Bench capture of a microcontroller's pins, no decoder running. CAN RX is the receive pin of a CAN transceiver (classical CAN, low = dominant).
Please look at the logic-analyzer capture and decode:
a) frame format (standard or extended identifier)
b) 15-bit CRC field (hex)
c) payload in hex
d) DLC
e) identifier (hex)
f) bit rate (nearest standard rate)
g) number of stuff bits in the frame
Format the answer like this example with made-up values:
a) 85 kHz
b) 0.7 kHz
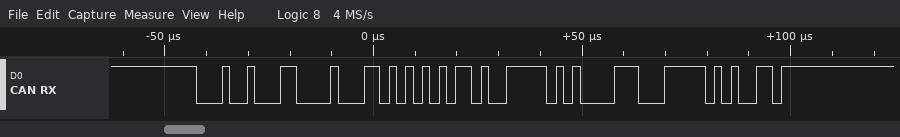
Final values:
a) standard
b) 0x47E9
c) 6A AD 3F 43
d) 4
e) 0x123
f) 500 kbit/s
g) 2
